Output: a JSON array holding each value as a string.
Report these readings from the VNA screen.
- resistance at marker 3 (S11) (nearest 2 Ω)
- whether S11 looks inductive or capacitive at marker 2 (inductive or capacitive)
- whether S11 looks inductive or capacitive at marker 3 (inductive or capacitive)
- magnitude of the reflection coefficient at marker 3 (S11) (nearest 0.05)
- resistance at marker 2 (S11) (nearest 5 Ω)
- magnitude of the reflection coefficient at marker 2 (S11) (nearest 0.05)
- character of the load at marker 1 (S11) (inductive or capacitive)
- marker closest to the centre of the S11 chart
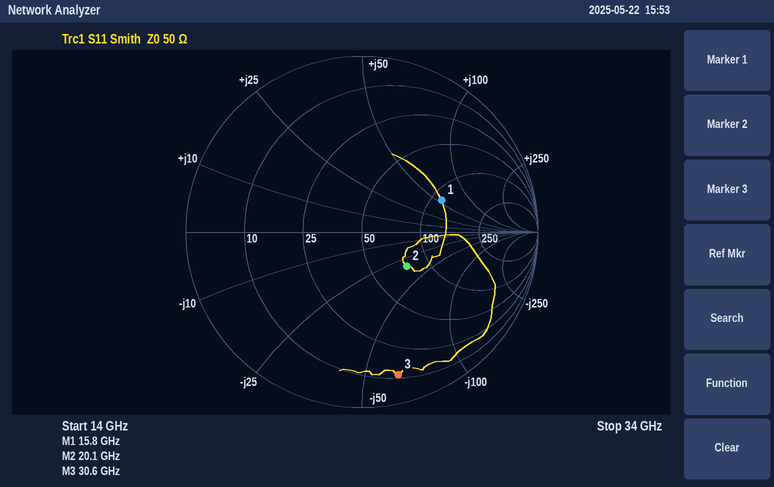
["12 Ω", "capacitive", "capacitive", "0.85", "75 Ω", "0.30", "inductive", "marker 2"]
